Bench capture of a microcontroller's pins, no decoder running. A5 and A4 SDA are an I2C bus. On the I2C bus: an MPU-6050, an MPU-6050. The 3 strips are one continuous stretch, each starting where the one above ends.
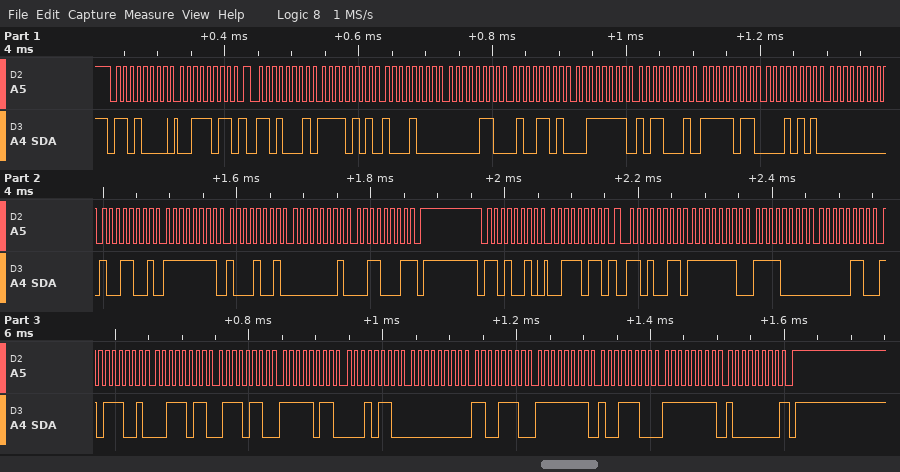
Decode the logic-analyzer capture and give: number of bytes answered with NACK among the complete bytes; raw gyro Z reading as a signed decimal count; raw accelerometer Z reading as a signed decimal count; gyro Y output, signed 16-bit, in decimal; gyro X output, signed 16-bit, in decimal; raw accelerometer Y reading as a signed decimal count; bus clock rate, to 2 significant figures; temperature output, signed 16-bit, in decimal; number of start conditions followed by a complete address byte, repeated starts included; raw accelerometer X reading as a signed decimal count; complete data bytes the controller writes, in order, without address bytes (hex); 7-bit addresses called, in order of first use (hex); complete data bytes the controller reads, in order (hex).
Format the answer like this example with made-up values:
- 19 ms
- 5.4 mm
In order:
- 2
- 305
- 16305
- -119
- 153
- 1613
- 100 kHz
- -1259
- 4
- -2680
- 3B 3B
- 0x68 0x69
- F5 88 06 4D 3F B1 FB 15 00 99 FF 89 01 31 FE F0 06 B9 3B 76 FB 16 00 CE FF 9C FF 80
